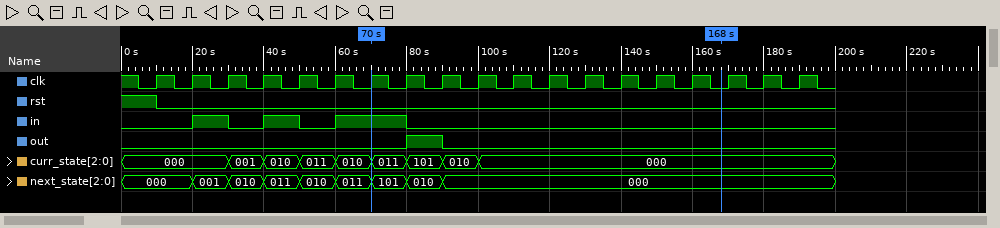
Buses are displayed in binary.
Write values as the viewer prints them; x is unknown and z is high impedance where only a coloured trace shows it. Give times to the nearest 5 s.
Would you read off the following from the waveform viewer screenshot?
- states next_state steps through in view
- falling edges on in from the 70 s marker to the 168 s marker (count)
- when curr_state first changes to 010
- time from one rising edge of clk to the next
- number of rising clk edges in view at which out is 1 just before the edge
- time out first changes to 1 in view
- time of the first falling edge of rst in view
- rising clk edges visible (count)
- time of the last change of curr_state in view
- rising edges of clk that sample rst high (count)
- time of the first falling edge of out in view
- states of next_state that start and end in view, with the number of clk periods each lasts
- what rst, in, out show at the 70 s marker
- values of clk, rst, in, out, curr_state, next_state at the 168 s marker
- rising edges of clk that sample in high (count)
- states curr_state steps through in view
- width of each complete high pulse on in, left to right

000, 001, 010, 011, 010, 011, 101, 010, 000
1
40 s
10 s
1
80 s
10 s
19
100 s
1
90 s
001: 1, 010: 1, 011: 1, 010: 1, 011: 1, 101: 1, 010: 1
rst=0, in=1, out=0
clk=0, rst=0, in=0, out=0, curr_state=000, next_state=000
4
000, 001, 010, 011, 010, 011, 101, 010, 000
10 s, 10 s, 20 s
